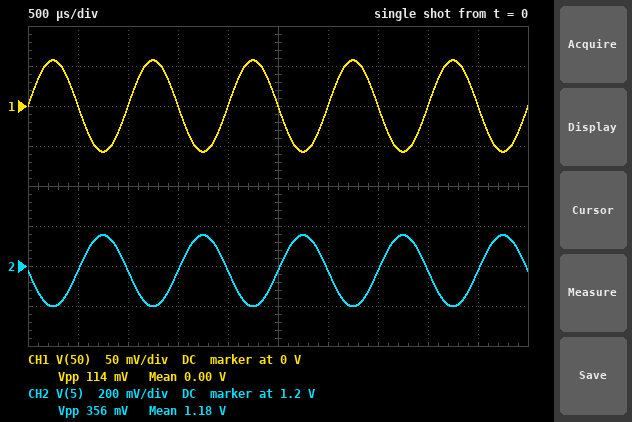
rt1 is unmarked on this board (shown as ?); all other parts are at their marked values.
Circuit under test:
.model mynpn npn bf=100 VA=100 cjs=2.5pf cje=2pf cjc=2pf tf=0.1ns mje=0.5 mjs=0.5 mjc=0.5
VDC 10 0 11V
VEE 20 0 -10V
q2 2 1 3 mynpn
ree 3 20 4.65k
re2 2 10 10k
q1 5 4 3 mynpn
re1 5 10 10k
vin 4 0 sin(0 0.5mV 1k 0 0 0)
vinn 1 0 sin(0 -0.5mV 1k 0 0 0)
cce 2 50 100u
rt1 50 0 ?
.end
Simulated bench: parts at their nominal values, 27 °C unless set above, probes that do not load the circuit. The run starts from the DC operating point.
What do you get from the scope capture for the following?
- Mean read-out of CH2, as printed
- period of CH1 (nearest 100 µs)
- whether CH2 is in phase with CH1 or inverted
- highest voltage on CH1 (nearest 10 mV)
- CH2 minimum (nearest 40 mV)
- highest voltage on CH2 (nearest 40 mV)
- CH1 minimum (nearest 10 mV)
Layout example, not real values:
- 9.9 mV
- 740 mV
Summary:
- 1.18 V
- 1.0 ms
- inverted
- 60 mV
- 1.00 V
- 1.36 V
- -60 mV
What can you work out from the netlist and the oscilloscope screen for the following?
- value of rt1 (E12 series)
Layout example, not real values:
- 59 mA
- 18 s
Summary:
- 4.7 kΩ
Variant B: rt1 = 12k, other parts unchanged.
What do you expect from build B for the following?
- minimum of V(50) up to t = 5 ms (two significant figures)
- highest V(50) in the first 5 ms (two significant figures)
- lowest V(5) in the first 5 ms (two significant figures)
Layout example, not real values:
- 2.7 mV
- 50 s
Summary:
- -96 mV
- 96 mV
- 1.0 V
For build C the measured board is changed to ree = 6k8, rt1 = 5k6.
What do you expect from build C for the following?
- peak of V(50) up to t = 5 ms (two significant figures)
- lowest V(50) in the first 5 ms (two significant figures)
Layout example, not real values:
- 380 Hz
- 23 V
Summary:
- 45 mV
- -45 mV
